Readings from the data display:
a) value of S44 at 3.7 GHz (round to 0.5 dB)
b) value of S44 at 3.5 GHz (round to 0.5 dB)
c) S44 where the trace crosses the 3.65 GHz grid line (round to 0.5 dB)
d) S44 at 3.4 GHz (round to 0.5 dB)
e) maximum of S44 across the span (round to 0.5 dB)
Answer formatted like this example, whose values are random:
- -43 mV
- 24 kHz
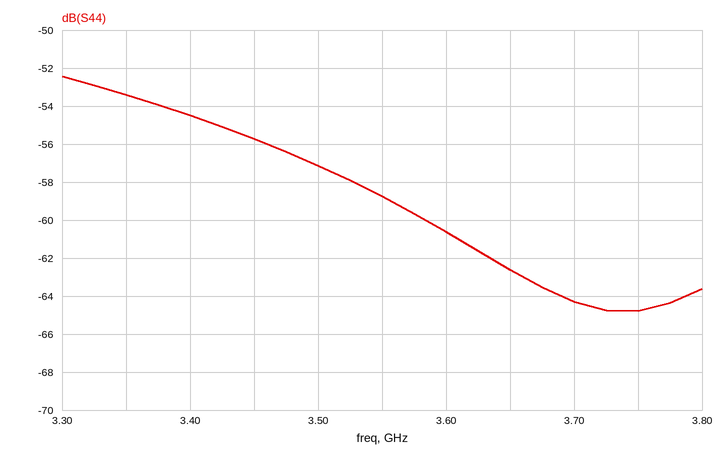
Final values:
- -64.5 dB
- -57.0 dB
- -62.5 dB
- -54.5 dB
- -52.5 dB
